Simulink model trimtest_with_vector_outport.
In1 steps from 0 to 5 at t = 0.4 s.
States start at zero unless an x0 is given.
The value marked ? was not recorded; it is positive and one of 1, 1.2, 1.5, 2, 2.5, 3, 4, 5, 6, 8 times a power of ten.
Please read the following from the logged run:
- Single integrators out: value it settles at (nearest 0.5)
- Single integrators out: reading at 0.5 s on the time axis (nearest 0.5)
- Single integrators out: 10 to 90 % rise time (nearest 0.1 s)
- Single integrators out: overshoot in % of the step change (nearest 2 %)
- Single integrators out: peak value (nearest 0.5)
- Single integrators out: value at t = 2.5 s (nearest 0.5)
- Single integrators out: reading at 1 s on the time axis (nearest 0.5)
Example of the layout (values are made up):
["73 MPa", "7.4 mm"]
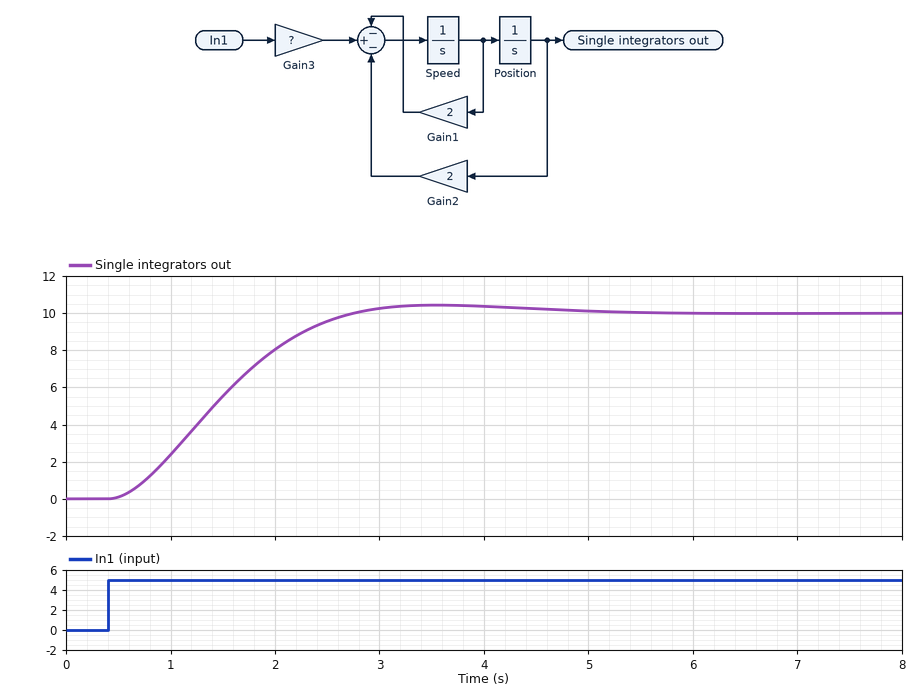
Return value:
["10.0", "0.0", "1.5 s", "4 %", "10.5", "9.5", "2.5"]
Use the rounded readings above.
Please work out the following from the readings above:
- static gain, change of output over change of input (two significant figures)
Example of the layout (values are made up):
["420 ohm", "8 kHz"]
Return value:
["2.0"]
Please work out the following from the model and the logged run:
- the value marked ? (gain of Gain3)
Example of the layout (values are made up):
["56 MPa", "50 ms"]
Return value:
["4"]
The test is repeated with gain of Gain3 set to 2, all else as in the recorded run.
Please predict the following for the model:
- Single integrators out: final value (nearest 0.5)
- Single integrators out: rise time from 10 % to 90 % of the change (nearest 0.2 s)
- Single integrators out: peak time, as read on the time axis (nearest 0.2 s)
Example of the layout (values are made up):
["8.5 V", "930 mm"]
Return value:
["5.0", "1.6 s", "3.6 s"]
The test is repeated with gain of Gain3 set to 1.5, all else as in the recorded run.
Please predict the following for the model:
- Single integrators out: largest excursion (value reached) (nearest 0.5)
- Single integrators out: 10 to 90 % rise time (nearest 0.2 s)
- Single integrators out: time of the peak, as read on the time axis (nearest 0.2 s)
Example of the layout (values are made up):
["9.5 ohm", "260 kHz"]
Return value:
["4.0", "1.6 s", "3.6 s"]
